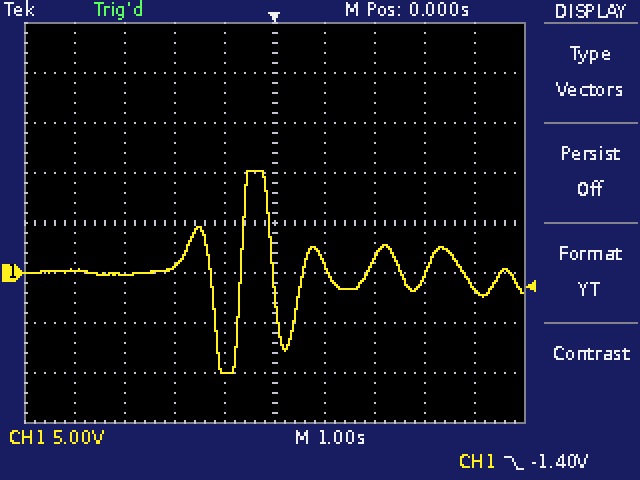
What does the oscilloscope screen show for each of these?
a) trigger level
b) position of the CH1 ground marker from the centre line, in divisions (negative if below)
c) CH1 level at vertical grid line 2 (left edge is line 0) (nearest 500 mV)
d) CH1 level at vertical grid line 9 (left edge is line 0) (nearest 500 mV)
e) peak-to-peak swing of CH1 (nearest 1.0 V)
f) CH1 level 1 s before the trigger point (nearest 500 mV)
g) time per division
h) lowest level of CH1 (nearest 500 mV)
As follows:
-1.40 V
-1.0 div
0.0 V
-1.5 V
20.0 V
-10.0 V
1 s
-10.0 V
